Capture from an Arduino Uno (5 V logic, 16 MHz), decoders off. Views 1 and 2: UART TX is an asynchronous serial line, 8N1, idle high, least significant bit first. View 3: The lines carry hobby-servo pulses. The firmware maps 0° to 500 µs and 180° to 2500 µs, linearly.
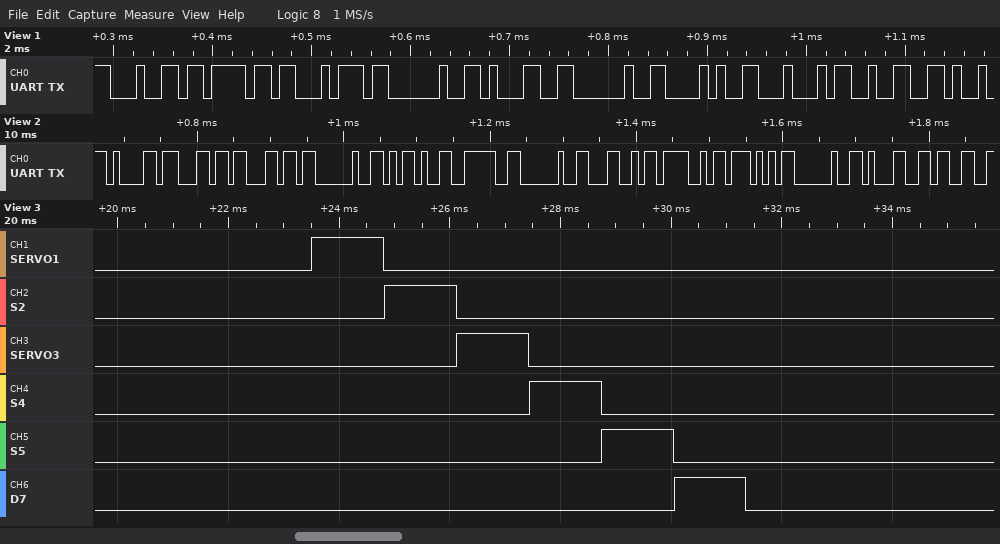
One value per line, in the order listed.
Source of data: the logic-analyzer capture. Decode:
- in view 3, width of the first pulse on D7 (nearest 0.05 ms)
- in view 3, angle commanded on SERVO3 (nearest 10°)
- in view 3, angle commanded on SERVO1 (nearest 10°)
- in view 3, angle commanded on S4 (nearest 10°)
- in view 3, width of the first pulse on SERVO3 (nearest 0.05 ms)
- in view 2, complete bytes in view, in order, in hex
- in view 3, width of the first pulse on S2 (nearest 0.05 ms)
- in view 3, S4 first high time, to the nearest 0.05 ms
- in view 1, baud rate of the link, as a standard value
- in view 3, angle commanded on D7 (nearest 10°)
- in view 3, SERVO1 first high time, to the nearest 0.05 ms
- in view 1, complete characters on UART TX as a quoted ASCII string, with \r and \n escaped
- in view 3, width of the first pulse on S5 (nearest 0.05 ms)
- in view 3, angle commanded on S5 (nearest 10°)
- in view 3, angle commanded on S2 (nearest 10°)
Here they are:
1.30 ms
70°
70°
70°
1.30 ms
61 6C 6C 20 2D 3E 20 4C 4F 57 20 31 33
1.30 ms
1.30 ms
115200 baud
70°
1.30 ms
"dot 1 (D2"
1.30 ms
70°
70°
